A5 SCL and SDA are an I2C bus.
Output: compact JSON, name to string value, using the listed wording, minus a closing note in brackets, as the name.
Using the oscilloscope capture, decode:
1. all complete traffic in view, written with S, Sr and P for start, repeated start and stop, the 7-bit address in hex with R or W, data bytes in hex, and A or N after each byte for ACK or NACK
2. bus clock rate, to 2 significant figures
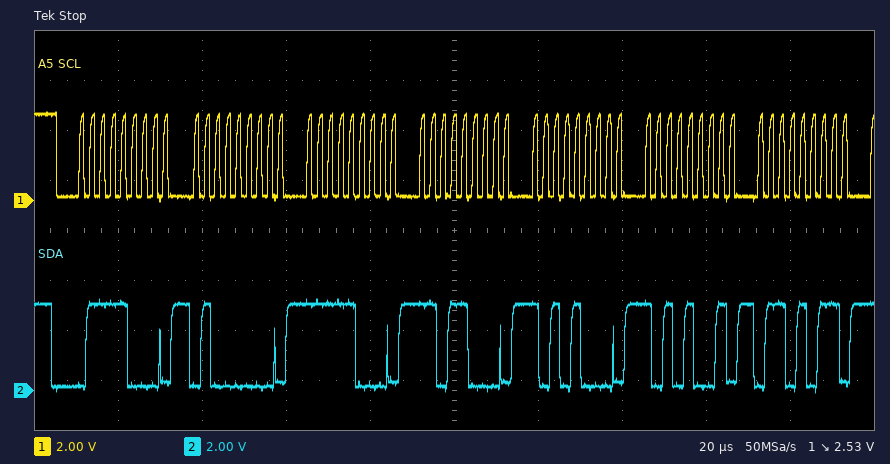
{"all complete traffic in view, written with S, Sr and P for start, repeated start and stop, the 7-bit address in hex with R or W, data bytes in hex, and A or N after each byte for ACK or NACK": "S 3CW A 40 A F8 A D8 A A8 A A9 A 6B A", "bus clock rate, to 2 significant figures": "400 kHz"}
